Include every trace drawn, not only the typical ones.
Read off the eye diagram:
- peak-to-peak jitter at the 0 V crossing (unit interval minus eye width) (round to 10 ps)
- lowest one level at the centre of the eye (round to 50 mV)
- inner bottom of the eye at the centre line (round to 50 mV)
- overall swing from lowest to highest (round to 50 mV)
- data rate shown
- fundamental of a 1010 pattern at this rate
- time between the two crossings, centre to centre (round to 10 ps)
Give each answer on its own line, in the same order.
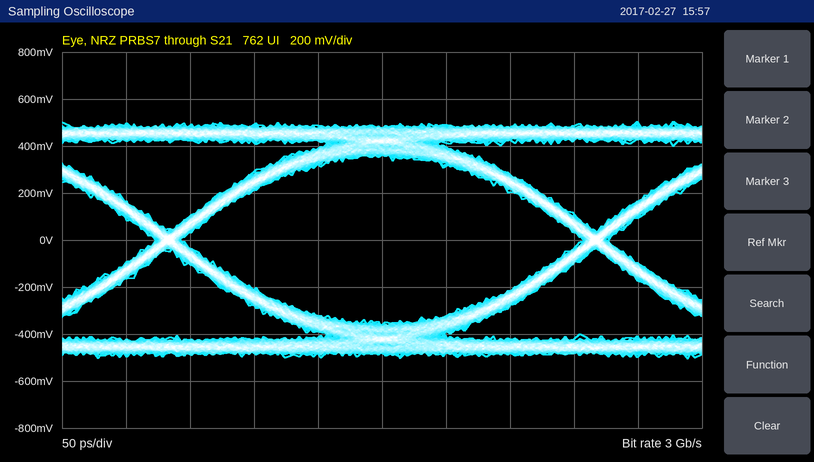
20 ps
350 mV
-350 mV
1.00 V
3 Gb/s
1.5 GHz
330 ps
